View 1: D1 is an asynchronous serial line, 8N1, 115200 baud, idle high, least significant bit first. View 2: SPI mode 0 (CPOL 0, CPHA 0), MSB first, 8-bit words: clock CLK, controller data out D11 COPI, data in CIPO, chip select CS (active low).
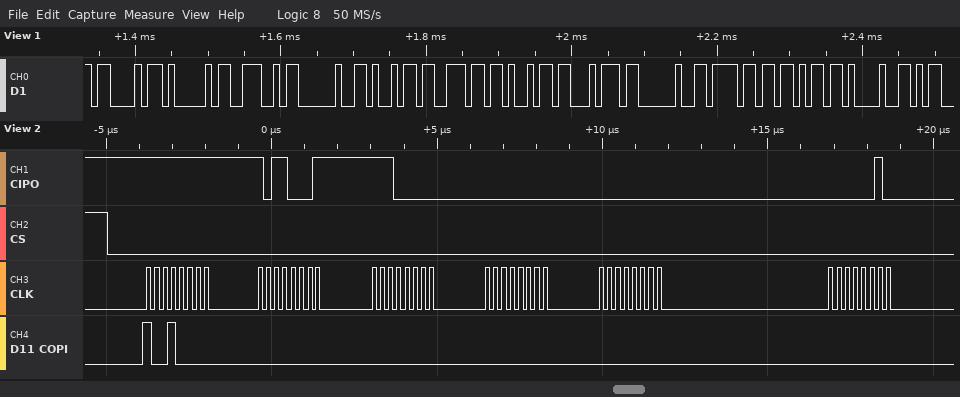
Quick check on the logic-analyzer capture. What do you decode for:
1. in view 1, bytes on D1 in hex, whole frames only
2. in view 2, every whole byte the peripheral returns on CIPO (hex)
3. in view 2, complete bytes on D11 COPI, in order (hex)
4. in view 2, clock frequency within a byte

43 41 4E 20 69 6E 69 74 20 6F 6B 21
FF B1 E0 00 00 02
90 00 00 00 00 00
4 MHz
